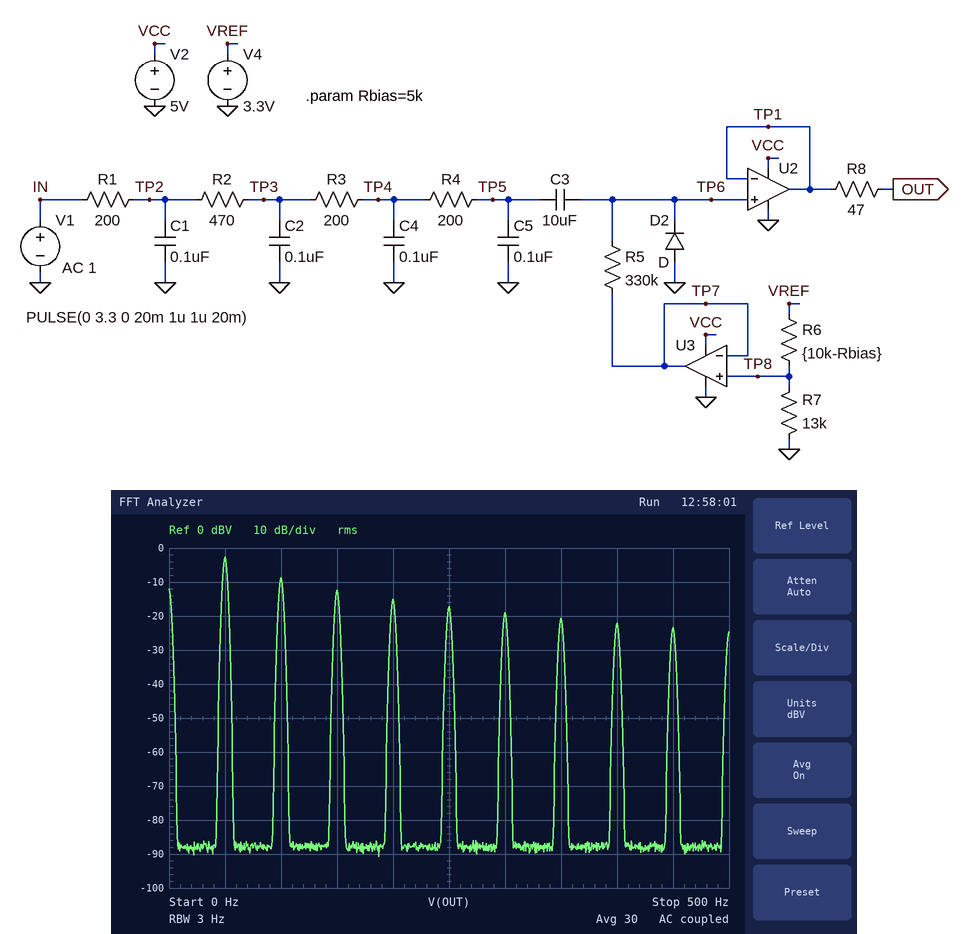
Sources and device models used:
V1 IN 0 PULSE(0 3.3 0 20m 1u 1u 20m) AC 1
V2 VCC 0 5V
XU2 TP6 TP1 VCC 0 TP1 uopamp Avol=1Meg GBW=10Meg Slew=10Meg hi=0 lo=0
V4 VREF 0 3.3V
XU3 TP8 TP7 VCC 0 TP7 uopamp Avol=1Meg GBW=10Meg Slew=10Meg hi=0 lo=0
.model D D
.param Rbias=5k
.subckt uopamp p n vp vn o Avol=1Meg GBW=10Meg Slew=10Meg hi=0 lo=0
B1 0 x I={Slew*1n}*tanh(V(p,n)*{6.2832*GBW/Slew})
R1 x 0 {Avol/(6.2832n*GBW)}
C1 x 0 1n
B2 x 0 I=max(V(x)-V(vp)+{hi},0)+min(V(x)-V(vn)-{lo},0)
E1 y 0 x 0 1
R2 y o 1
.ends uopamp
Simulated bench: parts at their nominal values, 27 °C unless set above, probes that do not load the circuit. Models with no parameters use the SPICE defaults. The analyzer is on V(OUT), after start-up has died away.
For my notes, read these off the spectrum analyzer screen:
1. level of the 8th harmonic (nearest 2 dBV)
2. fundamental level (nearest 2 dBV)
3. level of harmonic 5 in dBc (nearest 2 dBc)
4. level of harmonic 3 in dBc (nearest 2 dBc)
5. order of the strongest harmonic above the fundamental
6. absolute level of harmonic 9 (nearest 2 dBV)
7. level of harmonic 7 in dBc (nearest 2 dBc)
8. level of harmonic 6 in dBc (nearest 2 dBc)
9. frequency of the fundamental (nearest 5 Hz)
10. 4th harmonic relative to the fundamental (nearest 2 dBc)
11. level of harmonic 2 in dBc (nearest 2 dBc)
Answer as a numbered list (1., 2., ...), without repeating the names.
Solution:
1. -22 dBV
2. -2 dBV
3. -14 dBc
4. -10 dBc
5. 2
6. -24 dBV
7. -18 dBc
8. -16 dBc
9. 50 Hz
10. -12 dBc
11. -6 dBc
